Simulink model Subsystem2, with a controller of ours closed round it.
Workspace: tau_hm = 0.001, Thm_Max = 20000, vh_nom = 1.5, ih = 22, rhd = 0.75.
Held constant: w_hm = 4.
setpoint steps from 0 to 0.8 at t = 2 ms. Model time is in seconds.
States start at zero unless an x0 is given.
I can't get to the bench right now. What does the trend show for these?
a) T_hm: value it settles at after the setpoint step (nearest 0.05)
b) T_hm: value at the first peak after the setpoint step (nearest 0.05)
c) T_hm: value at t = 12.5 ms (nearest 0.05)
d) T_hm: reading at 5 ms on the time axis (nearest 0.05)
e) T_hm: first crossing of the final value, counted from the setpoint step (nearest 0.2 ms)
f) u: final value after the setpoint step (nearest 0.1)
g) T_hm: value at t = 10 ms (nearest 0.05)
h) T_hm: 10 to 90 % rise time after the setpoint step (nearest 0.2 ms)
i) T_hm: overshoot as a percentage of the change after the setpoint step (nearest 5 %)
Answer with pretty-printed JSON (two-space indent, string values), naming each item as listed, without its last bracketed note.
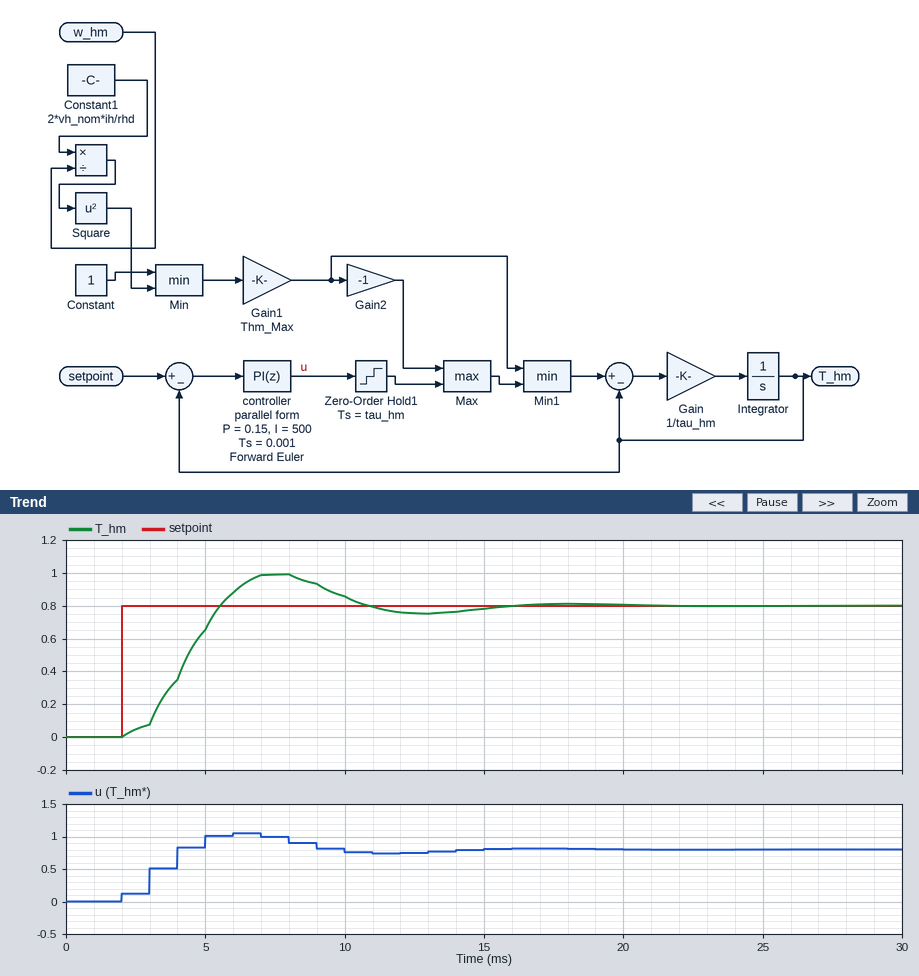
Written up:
{
  "T_hm: value it settles at after the setpoint step": "0.80",
  "T_hm: value at the first peak after the setpoint step": "1.00",
  "T_hm: value at t = 12.5 ms": "0.75",
  "T_hm: reading at 5 ms on the time axis": "0.65",
  "T_hm: first crossing of the final value, counted from the setpoint step": "3.6 ms",
  "u: final value after the setpoint step": "0.8",
  "T_hm: value at t = 10 ms": "0.85",
  "T_hm: 10 to 90 % rise time after the setpoint step": "2.2 ms",
  "T_hm: overshoot as a percentage of the change after the setpoint step": "25 %"
}
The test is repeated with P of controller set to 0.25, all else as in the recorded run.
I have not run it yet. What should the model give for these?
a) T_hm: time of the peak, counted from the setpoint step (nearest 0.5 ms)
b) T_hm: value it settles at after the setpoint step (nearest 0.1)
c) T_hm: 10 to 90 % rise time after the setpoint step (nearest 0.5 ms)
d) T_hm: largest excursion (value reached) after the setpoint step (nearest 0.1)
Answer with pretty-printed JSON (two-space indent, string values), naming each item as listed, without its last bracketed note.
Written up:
{
  "T_hm: time of the peak, counted from the setpoint step": "5.0 ms",
  "T_hm: value it settles at after the setpoint step": "0.8",
  "T_hm: 10 to 90 % rise time after the setpoint step": "2.5 ms",
  "T_hm: largest excursion (value reached) after the setpoint step": "0.9"
}
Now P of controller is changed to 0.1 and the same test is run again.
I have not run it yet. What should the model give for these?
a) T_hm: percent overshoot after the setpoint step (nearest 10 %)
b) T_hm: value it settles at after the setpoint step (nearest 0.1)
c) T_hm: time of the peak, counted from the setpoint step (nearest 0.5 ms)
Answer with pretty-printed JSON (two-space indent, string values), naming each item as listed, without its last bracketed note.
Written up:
{
  "T_hm: percent overshoot after the setpoint step": "30 %",
  "T_hm: value it settles at after the setpoint step": "0.8",
  "T_hm: time of the peak, counted from the setpoint step": "6.0 ms"
}
